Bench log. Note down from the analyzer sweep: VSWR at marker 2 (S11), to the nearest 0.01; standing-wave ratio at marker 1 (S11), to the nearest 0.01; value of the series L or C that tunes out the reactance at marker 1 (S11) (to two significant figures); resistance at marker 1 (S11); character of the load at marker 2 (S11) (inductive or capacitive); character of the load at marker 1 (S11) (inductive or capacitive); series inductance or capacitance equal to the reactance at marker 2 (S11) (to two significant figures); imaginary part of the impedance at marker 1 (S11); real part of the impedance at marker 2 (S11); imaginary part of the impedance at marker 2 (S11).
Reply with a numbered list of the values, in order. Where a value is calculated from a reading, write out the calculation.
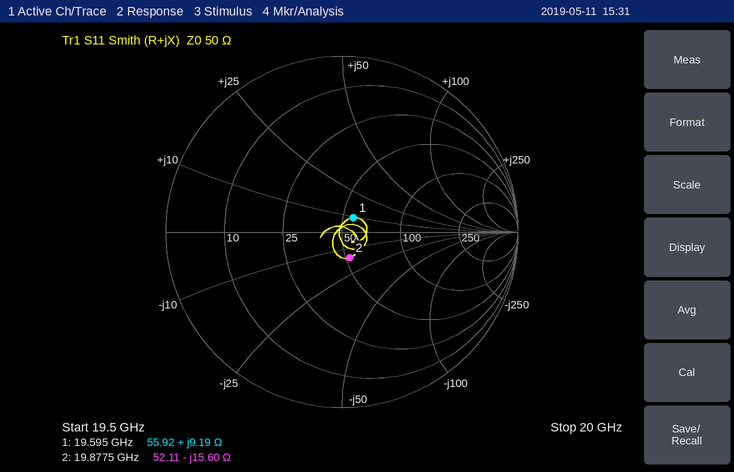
1. 1.36
2. 1.23
3. C = 1/(2π × 19.595 GHz × 9.19 Ω) ≈ 884 fF, so 880 fF to two significant figures
4. 55.92 Ω
5. capacitive
6. inductive
7. C = 1/(2π × 19.8775 GHz × 15.6 Ω) ≈ 513 fF, so 510 fF to two significant figures
8. +9.19 Ω
9. 52.11 Ω
10. -15.60 Ω
